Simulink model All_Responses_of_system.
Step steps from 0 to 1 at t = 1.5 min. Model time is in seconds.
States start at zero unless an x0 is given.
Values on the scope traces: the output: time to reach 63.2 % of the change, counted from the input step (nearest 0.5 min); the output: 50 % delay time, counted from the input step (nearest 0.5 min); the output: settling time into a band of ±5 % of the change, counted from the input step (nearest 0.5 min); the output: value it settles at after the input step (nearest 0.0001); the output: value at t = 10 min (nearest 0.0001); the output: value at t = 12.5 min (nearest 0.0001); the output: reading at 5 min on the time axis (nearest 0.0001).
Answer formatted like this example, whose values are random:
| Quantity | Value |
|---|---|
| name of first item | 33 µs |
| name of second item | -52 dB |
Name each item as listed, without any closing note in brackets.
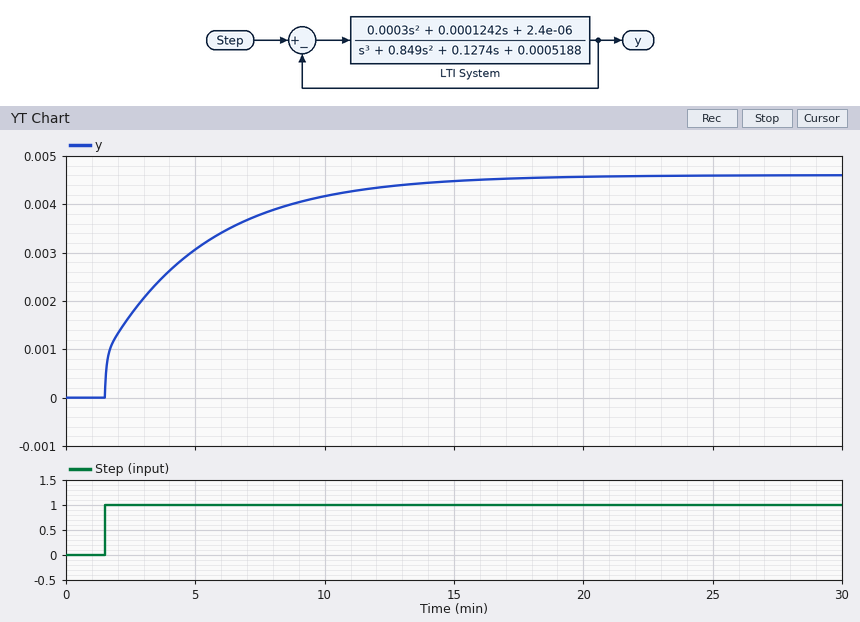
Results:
| Quantity | Value |
|---|---|
| the output: time to reach 63.2 % of the change, counted from the input step | 3.0 min |
| the output: 50 % delay time, counted from the input step | 2.0 min |
| the output: settling time into a band of ±5 % of the change, counted from the input step | 11.0 min |
| the output: value it settles at after the input step | 0.0046 |
| the output: value at t = 10 min | 0.0042 |
| the output: value at t = 12.5 min | 0.0044 |
| the output: reading at 5 min on the time axis | 0.0031 |
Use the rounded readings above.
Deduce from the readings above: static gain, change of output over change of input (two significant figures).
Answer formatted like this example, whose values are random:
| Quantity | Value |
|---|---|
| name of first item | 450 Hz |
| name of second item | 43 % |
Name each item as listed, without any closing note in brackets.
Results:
| Quantity | Value |
|---|---|
| static gain, change of output over change of input | 0.0046 |
